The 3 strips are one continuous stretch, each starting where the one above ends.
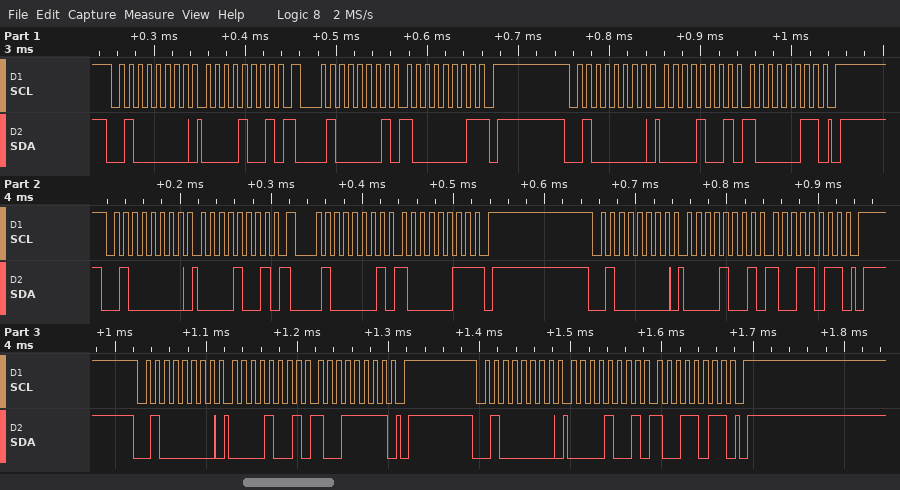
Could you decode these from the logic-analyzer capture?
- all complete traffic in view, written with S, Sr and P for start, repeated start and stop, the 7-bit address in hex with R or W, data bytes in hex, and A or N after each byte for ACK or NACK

S 20W A 09 A Sr 20R A 81 N P S 20W A 09 A 83 A P S 20W A 09 A Sr 20R A 83 N P S 20W A 09 A 9B A P S 20W A 09 A 9F A P S 20W A 09 A 9B A P
